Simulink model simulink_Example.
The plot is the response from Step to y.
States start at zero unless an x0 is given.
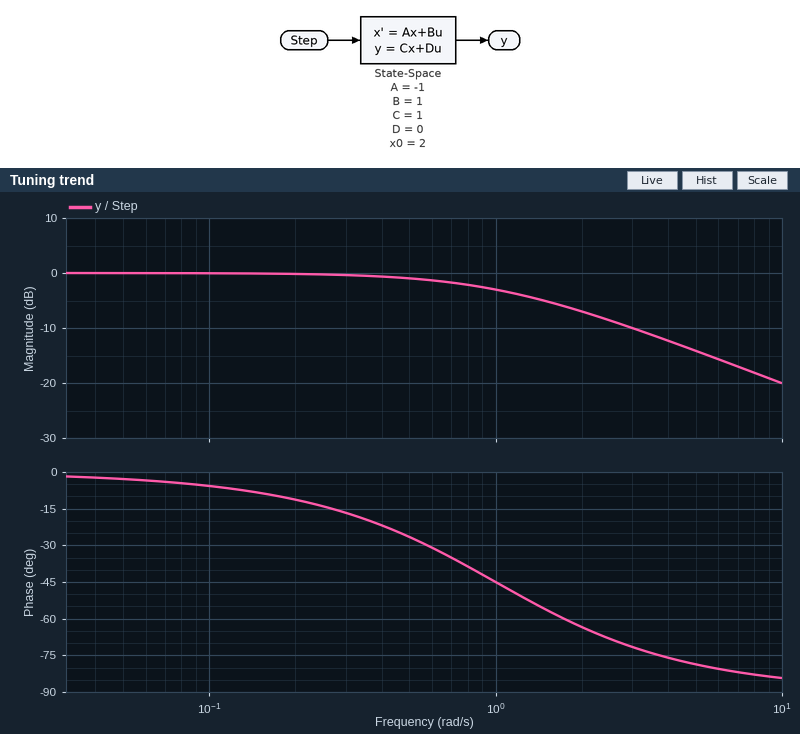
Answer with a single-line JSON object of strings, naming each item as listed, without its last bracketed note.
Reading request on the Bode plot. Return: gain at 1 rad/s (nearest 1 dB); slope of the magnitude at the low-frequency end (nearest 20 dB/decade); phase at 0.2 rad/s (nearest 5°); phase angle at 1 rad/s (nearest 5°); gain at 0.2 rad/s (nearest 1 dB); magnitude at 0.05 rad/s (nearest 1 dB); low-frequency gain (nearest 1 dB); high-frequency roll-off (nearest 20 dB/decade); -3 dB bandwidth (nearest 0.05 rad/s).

{"gain at 1 rad/s": "-3 dB", "slope of the magnitude at the low-frequency end": "0 dB/decade", "phase at 0.2 rad/s": "-10°", "phase angle at 1 rad/s": "-45°", "gain at 0.2 rad/s": "0 dB", "magnitude at 0.05 rad/s": "0 dB", "low-frequency gain": "0 dB", "high-frequency roll-off": "-20 dB/decade", "-3 dB bandwidth": "1.00 rad/s"}
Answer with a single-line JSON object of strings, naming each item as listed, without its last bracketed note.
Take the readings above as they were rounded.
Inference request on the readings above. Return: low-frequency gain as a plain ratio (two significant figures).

{"low-frequency gain as a plain ratio": "1.0"}
